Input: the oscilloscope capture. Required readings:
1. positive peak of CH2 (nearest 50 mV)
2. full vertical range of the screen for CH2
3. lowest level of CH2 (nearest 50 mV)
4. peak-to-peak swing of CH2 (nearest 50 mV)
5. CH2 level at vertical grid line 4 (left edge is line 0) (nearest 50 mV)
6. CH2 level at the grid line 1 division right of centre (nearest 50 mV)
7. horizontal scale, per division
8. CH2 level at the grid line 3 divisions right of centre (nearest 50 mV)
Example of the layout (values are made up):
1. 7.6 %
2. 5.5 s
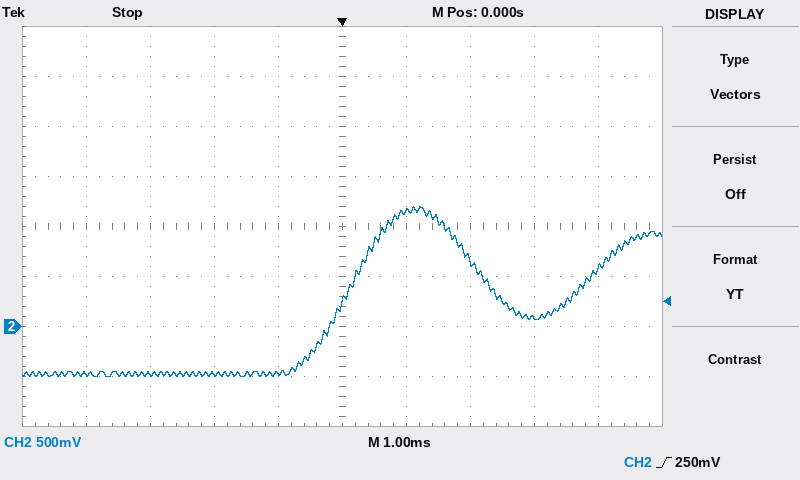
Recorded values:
1. 1.20 V
2. 4 V
3. -500 mV
4. 1.70 V
5. -450 mV
6. 1.15 V
7. 1 ms
8. 100 mV
